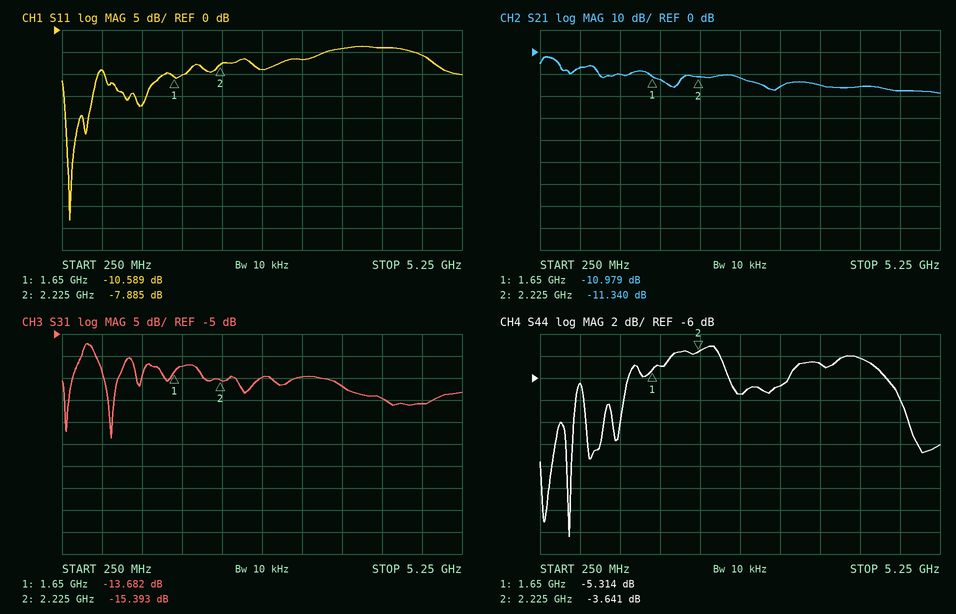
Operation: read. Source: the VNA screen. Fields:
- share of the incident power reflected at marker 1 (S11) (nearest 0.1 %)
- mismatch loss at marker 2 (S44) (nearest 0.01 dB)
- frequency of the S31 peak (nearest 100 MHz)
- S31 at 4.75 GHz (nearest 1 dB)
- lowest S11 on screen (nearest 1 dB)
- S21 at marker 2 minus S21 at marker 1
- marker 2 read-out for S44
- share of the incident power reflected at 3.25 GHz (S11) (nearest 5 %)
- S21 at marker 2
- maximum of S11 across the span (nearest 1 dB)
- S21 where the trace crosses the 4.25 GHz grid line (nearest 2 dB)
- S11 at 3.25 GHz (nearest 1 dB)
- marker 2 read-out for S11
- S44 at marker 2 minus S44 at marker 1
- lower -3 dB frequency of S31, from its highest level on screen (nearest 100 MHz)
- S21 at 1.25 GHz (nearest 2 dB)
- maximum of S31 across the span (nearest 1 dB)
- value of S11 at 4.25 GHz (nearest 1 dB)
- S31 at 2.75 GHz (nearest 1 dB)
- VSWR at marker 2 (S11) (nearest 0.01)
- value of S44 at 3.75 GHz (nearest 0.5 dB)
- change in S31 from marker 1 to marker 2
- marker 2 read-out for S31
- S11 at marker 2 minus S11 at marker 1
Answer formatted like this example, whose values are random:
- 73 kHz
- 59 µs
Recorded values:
- 8.7 %
- 2.46 dB
- 600 MHz
- -21 dB
- -43 dB
- -0.361 dB
- -3.641 dB
- 20 %
- -11.340 dB
- -4 dB
- -16 dB
- -7 dB
- -7.885 dB
- 1.673 dB
- 500 MHz
- -10 dB
- -7 dB
- -4 dB
- -15 dB
- 2.35
- -4.5 dB
- -1.711 dB
- -15.393 dB
- 2.704 dB
